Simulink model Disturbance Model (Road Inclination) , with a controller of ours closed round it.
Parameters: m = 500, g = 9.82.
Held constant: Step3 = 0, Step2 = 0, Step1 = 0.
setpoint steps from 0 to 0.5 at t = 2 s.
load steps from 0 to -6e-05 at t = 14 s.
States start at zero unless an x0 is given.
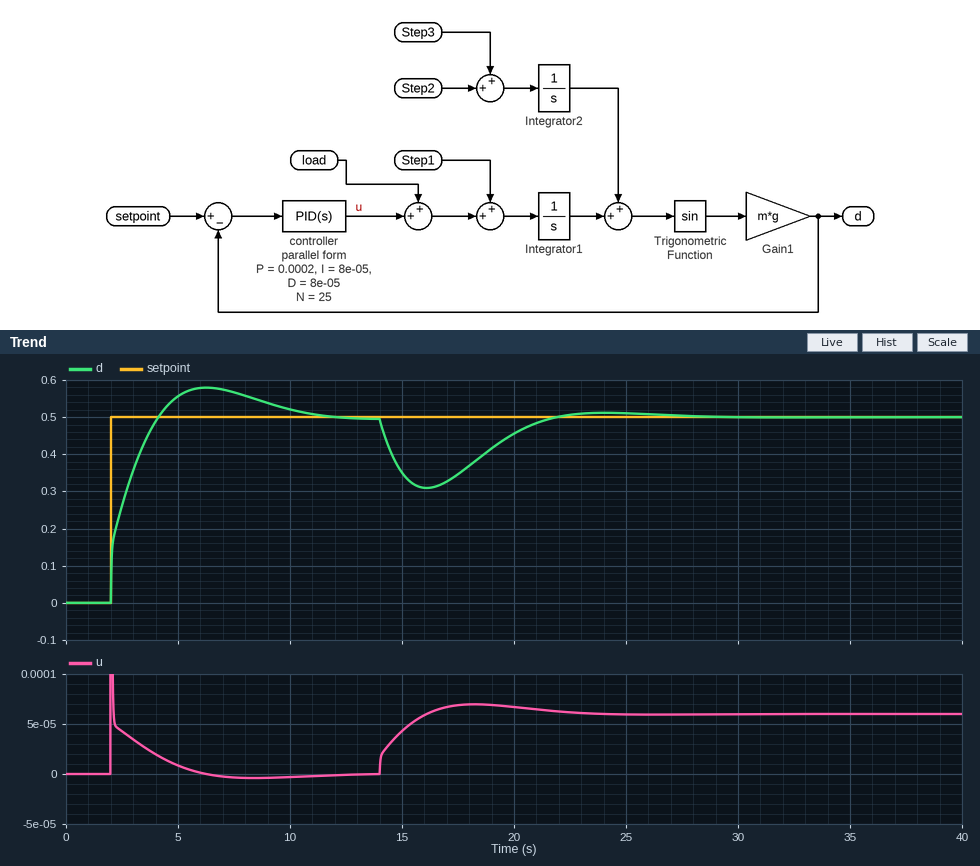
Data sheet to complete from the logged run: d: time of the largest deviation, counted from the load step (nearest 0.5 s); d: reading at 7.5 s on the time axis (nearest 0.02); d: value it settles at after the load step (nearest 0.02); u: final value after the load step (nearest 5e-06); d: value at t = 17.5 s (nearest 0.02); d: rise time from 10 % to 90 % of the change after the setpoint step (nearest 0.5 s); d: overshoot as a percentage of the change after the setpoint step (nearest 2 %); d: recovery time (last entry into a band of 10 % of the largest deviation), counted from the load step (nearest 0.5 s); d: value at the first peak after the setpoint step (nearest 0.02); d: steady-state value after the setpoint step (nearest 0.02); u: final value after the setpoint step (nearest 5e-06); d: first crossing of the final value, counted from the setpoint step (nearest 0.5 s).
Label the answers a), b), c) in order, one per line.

a) 2.0 s
b) 0.56
c) 0.50
d) 0.000060
e) 0.34
f) 1.5 s
g) 16 %
h) 7.0 s
i) 0.58
j) 0.50
k) 0.000000
l) 2.0 s
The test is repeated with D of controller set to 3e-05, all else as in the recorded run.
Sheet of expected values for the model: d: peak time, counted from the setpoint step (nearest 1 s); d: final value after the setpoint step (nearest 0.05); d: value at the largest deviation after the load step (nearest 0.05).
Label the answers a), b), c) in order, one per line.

a) 4 s
b) 0.50
c) 0.30
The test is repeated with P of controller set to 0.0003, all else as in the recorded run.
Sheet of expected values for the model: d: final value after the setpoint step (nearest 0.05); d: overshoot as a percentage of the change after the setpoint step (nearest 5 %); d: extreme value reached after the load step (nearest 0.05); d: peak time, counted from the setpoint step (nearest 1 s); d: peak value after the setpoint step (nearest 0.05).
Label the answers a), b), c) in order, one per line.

a) 0.50
b) 10 %
c) 0.35
d) 4 s
e) 0.55
